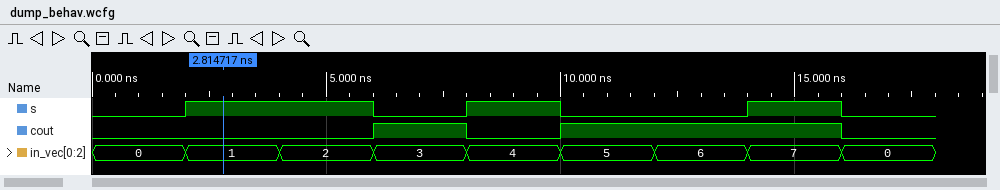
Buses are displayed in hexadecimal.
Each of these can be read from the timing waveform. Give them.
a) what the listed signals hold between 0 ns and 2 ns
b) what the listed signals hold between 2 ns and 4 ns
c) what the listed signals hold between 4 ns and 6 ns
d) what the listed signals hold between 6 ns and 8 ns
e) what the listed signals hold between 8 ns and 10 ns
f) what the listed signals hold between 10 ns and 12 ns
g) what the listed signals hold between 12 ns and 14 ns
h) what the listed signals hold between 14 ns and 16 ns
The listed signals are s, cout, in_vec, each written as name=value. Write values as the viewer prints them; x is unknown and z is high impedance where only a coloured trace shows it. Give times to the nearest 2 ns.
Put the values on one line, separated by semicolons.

s=0, cout=0, in_vec=0; s=1, cout=0, in_vec=1; s=1, cout=0, in_vec=2; s=0, cout=1, in_vec=3; s=1, cout=0, in_vec=4; s=0, cout=1, in_vec=5; s=0, cout=1, in_vec=6; s=1, cout=1, in_vec=7
